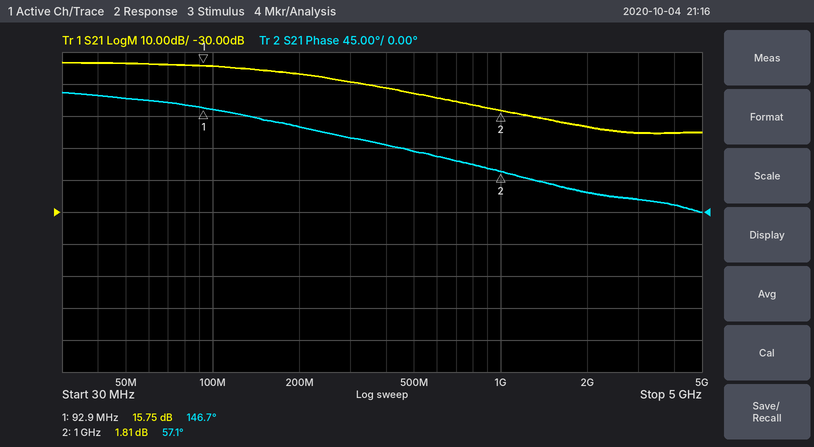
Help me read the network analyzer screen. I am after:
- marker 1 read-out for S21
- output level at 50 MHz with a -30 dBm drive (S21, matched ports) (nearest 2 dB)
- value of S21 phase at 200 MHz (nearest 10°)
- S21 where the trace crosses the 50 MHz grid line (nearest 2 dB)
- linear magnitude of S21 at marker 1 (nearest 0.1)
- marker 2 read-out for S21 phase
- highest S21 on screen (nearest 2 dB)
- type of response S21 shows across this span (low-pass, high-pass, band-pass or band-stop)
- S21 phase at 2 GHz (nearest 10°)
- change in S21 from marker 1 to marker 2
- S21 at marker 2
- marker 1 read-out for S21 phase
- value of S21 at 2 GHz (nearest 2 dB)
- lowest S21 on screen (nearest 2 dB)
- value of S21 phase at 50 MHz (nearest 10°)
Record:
15.75 dB
-14 dBm
120°
16 dB
6.1
57.1°
16 dB
low-pass
30°
-13.94 dB
1.81 dB
146.7°
-4 dB
-6 dB
160°
